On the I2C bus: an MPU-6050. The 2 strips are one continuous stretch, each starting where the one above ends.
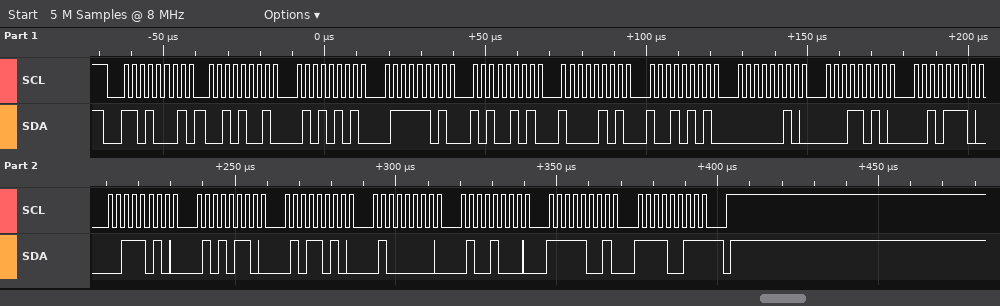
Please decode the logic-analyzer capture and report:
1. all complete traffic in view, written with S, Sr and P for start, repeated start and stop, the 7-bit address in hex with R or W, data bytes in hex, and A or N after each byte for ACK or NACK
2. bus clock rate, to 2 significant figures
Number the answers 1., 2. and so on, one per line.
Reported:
1. S 68R A 29 A 55 A 7D A A5 A 85 A 95 A 02 A 1A A 2E A 3A A 56 A 5A A 40 A 48 A F9 A F3 N P
2. 400 kHz
